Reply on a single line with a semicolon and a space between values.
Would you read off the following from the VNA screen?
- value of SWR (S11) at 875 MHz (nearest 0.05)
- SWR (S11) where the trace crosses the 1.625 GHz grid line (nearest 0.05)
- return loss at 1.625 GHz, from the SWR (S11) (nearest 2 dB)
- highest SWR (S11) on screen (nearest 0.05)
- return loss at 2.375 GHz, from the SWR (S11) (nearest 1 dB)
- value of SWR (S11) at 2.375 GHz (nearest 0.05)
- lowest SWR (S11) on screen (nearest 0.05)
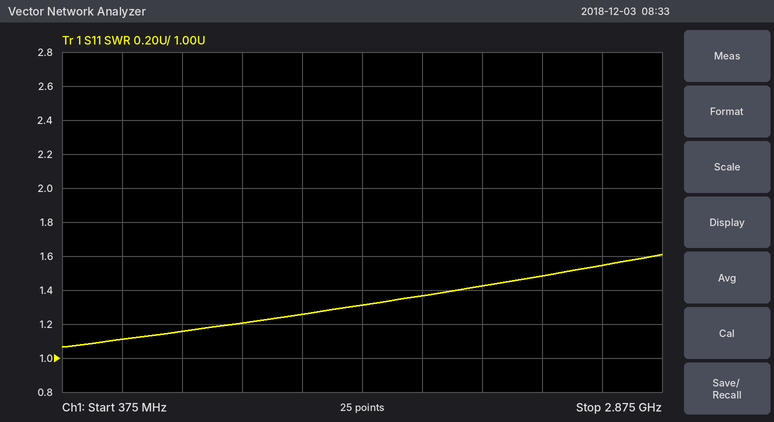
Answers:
1.15; 1.30; 18 dB; 1.60; 14 dB; 1.50; 1.05
